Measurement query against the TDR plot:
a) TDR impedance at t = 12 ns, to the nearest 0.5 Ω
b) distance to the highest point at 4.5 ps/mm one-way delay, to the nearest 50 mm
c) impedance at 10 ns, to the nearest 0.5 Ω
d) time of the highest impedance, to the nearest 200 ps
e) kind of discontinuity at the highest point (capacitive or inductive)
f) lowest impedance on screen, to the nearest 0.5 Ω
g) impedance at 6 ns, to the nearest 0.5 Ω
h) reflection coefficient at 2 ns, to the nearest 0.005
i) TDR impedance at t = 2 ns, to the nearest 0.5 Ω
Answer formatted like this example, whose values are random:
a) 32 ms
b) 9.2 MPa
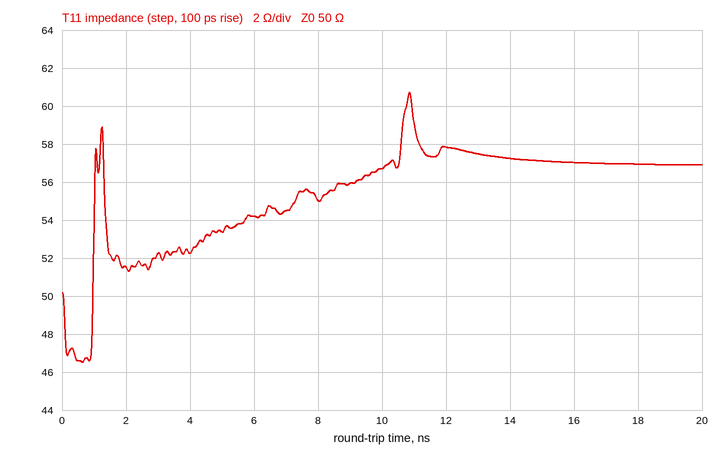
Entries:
a) 58.0 Ω
b) 1.20 m
c) 56.5 Ω
d) 10.8 ns
e) inductive
f) 46.5 Ω
g) 54.0 Ω
h) +0.015
i) 51.5 Ω
